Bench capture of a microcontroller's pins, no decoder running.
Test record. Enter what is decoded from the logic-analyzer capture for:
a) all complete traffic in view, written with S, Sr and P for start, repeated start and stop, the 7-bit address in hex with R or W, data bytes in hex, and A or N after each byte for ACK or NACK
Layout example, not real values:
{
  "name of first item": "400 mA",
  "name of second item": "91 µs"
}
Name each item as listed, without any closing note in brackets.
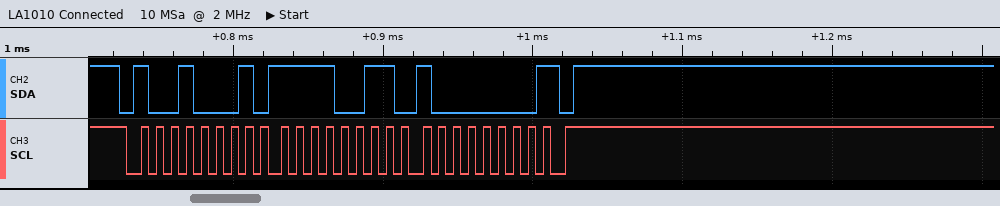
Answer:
{
  "all complete traffic in view, written with S, Sr and P for start, repeated start and stop, the 7-bit address in hex with R or W, data bytes in hex, and A or N after each byte for ACK or NACK": "S 48R A F3 A 80 N P"
}
